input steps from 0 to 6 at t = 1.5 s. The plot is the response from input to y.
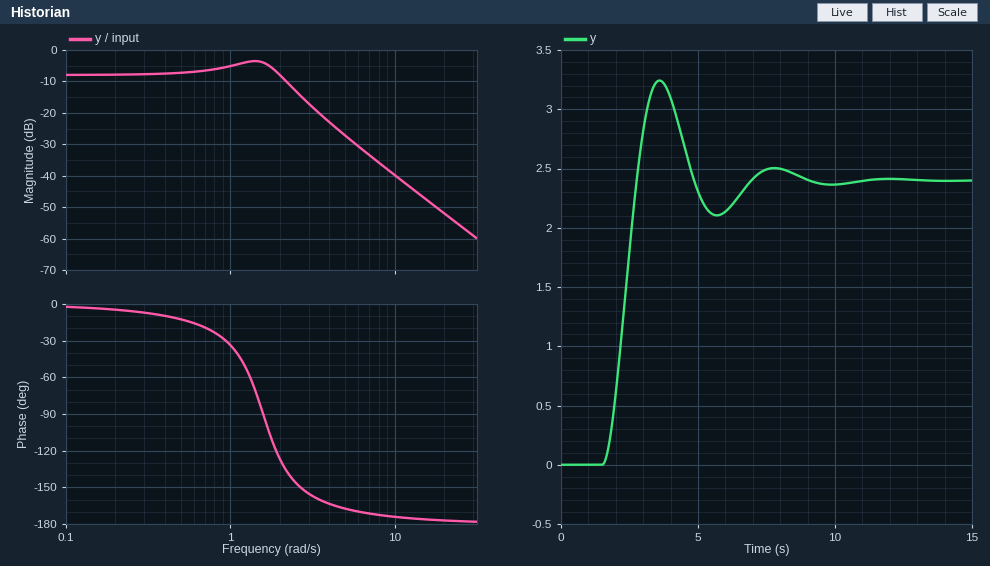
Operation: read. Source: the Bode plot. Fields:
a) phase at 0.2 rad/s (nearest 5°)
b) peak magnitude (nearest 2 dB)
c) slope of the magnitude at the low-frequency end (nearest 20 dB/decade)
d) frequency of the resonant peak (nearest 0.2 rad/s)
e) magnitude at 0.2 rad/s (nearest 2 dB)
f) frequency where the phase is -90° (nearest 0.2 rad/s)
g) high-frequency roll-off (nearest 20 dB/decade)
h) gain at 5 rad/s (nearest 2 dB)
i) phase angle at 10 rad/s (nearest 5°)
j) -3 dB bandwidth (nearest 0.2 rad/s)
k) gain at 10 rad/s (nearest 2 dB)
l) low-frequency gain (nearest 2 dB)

-5°
-4 dB
0 dB/decade
1.4 rad/s
-8 dB
1.6 rad/s
-40 dB/decade
-28 dB
-175°
2.2 rad/s
-40 dB
-8 dB
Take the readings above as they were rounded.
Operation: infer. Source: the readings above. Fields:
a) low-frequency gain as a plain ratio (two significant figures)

0.40
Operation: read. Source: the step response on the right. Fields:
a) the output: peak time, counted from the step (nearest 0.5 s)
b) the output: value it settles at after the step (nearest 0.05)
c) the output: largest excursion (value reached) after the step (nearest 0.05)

2.0 s
2.40
3.25
